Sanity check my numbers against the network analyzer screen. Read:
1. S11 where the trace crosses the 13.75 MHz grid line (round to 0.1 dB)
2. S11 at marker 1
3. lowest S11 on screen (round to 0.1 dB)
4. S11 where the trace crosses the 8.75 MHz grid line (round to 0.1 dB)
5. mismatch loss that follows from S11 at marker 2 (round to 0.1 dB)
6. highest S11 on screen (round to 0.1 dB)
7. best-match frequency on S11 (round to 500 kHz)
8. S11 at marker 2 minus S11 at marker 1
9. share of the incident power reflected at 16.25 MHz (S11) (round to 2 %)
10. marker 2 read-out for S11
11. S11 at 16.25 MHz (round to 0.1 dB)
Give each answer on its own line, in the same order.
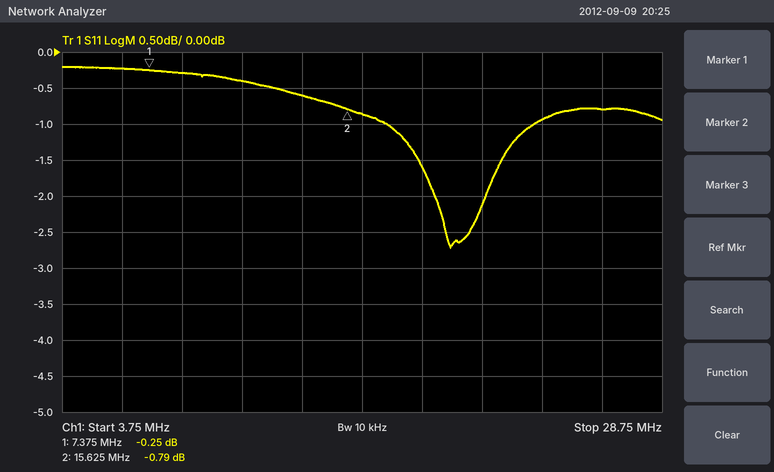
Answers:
-0.6 dB
-0.25 dB
-2.7 dB
-0.3 dB
7.8 dB
-0.2 dB
20.0 MHz
-0.54 dB
82 %
-0.79 dB
-0.9 dB
